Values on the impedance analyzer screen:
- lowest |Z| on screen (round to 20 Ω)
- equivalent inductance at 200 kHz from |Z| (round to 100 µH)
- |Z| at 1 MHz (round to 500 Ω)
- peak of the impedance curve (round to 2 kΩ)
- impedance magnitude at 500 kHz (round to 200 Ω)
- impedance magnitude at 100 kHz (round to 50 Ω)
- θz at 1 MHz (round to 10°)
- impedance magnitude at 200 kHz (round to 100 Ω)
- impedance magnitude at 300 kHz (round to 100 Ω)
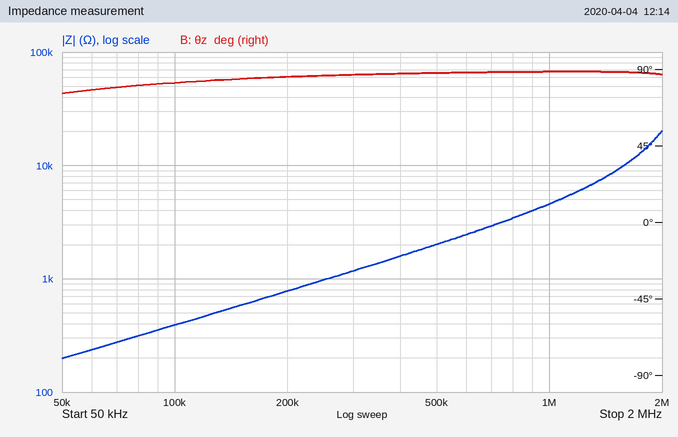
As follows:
200 Ω
600 µH
4.5 kΩ
20 kΩ
2.0 kΩ
400 Ω
90°
800 Ω
1.2 kΩ
